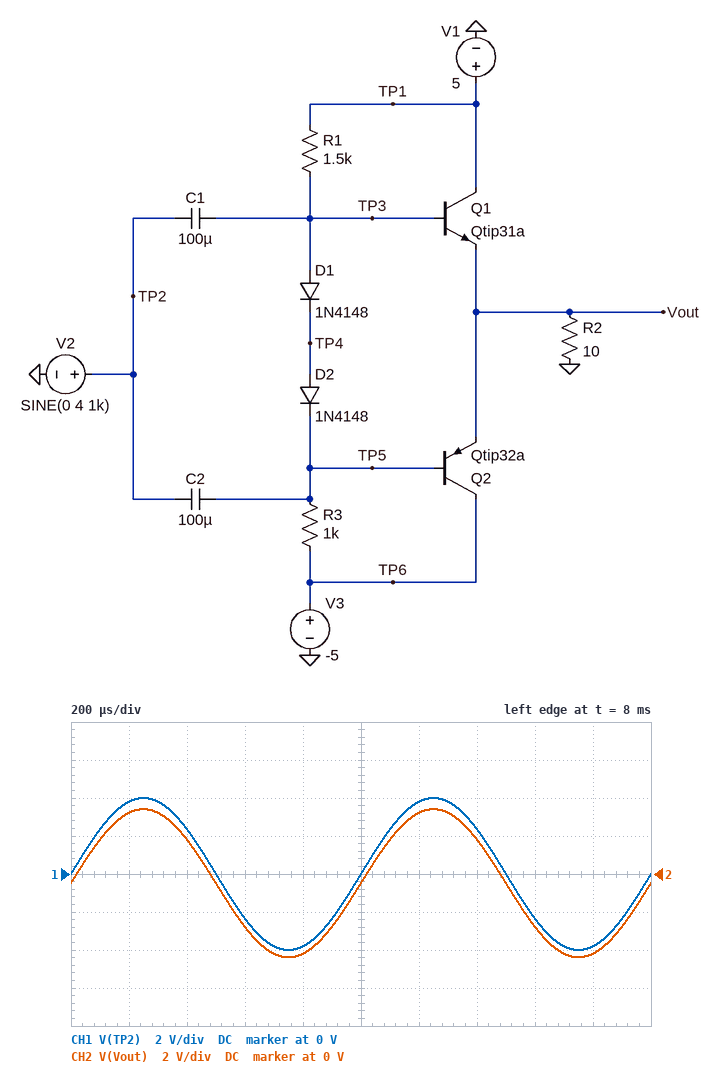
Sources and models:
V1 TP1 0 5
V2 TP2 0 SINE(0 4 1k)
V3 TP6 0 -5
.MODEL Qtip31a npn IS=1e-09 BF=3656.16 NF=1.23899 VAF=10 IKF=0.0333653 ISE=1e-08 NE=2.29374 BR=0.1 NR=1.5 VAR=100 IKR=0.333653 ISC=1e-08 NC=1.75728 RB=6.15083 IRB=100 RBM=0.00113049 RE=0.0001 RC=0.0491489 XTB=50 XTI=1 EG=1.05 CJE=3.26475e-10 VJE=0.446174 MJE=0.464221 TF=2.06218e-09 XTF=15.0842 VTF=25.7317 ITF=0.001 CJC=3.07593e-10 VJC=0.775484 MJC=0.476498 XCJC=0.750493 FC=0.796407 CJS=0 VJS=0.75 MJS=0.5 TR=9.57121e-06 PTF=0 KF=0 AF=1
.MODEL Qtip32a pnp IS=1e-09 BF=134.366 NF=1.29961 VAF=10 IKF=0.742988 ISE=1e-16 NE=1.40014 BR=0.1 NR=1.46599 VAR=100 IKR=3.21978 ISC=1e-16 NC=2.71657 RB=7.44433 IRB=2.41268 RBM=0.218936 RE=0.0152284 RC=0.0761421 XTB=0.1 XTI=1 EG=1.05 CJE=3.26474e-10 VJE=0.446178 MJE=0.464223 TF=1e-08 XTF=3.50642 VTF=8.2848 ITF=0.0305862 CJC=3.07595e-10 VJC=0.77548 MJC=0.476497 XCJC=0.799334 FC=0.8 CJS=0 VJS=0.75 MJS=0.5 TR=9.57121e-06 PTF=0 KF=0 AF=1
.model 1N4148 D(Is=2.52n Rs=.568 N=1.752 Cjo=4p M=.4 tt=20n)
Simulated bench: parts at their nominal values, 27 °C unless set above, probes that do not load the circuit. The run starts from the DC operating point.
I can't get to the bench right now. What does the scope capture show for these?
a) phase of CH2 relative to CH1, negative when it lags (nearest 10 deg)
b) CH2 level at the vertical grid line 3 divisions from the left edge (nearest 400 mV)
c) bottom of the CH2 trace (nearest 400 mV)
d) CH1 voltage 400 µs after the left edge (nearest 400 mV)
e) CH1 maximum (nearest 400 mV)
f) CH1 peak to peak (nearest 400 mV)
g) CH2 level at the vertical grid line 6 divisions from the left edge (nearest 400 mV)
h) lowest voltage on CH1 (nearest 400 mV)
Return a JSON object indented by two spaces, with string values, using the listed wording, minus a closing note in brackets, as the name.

{
  "phase of CH2 relative to CH1, negative when it lags": "0 deg",
  "CH2 level at the vertical grid line 3 divisions from the left edge": "-2.8 V",
  "bottom of the CH2 trace": "-4.4 V",
  "CH1 voltage 400 µs after the left edge": "2.4 V",
  "CH1 maximum": "4.0 V",
  "CH1 peak to peak": "8.0 V",
  "CH2 level at the vertical grid line 6 divisions from the left edge": "3.2 V",
  "lowest voltage on CH1": "-4.0 V"
}
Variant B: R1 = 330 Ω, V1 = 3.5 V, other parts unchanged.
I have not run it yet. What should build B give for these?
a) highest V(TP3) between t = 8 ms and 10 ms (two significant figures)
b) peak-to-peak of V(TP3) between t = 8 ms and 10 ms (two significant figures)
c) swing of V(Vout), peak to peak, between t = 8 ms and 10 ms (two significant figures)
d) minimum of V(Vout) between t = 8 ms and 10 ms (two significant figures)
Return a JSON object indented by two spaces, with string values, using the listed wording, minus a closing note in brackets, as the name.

{
  "highest V(TP3) between t = 8 ms and 10 ms": "4.6 V",
  "peak-to-peak of V(TP3) between t = 8 ms and 10 ms": "8.0 V",
  "swing of V(Vout), peak to peak, between t = 8 ms and 10 ms": "6.8 V",
  "minimum of V(Vout) between t = 8 ms and 10 ms": "-3.4 V"
}
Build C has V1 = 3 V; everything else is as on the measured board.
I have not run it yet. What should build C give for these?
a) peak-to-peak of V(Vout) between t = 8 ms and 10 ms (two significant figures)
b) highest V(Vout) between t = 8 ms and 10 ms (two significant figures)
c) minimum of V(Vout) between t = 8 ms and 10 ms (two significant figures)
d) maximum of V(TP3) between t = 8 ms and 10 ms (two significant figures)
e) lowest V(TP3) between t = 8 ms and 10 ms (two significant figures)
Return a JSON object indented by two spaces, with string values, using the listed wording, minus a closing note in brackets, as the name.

{
  "peak-to-peak of V(Vout) between t = 8 ms and 10 ms": "7.6 V",
  "highest V(Vout) between t = 8 ms and 10 ms": "2.8 V",
  "minimum of V(Vout) between t = 8 ms and 10 ms": "-4.8 V",
  "maximum of V(TP3) between t = 8 ms and 10 ms": "3.5 V",
  "lowest V(TP3) between t = 8 ms and 10 ms": "-4.5 V"
}
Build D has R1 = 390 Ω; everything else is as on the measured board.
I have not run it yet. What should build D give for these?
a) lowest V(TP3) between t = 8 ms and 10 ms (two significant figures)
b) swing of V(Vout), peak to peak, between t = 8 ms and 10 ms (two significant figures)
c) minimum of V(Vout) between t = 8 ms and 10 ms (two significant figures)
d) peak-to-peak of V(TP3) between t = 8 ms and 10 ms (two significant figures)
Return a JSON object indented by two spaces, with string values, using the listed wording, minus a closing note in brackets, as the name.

{
  "lowest V(TP3) between t = 8 ms and 10 ms": "-2.1 V",
  "swing of V(Vout), peak to peak, between t = 8 ms and 10 ms": "7.5 V",
  "minimum of V(Vout) between t = 8 ms and 10 ms": "-2.6 V",
  "peak-to-peak of V(TP3) between t = 8 ms and 10 ms": "8.0 V"
}
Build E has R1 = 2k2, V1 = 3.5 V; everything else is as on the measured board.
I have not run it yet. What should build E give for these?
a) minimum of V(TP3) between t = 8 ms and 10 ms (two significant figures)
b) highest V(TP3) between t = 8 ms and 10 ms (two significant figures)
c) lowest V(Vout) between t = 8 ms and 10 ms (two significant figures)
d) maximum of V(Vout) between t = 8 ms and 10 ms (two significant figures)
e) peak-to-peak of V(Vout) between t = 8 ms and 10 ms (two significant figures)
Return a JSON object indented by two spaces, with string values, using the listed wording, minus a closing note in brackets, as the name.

{
  "minimum of V(TP3) between t = 8 ms and 10 ms": "-4.7 V",
  "highest V(TP3) between t = 8 ms and 10 ms": "3.3 V",
  "lowest V(Vout) between t = 8 ms and 10 ms": "-4.8 V",
  "maximum of V(Vout) between t = 8 ms and 10 ms": "2.6 V",
  "peak-to-peak of V(Vout) between t = 8 ms and 10 ms": "7.4 V"
}
